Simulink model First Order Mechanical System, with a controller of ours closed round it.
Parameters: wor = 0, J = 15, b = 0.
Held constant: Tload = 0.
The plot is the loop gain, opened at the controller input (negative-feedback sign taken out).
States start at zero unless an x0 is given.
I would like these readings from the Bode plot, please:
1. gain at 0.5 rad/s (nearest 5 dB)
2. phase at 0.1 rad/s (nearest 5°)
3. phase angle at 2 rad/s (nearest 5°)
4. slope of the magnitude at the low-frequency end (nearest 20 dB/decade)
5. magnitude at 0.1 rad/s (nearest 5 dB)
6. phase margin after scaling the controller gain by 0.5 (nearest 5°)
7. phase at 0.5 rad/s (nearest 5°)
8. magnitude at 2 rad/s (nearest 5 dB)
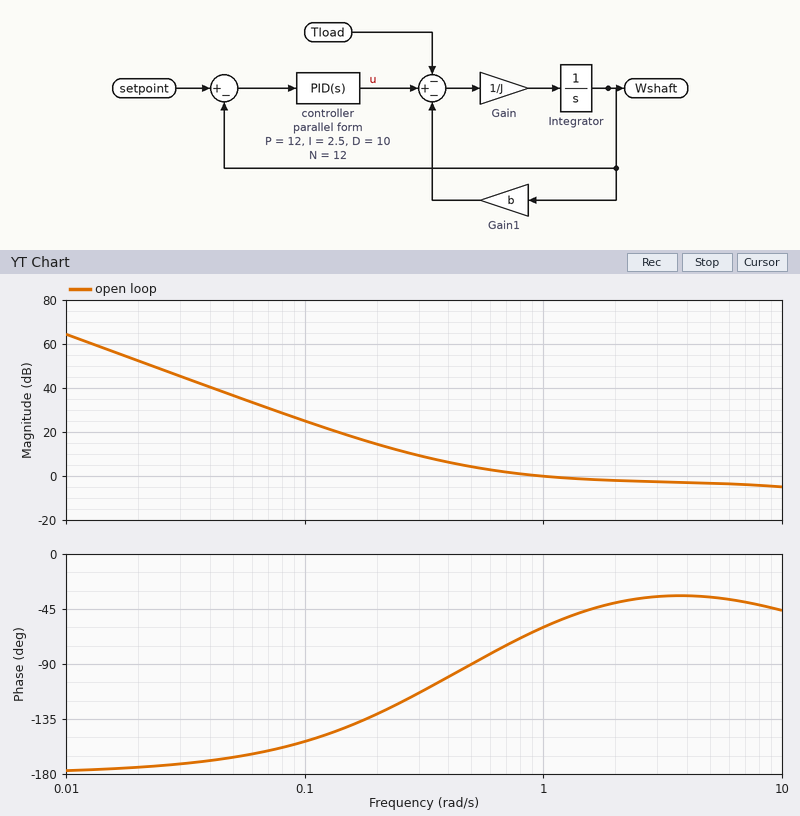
5 dB
-155°
-40°
-40 dB/decade
25 dB
80°
-90°
0 dB
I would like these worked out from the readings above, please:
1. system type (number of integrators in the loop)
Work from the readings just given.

2
